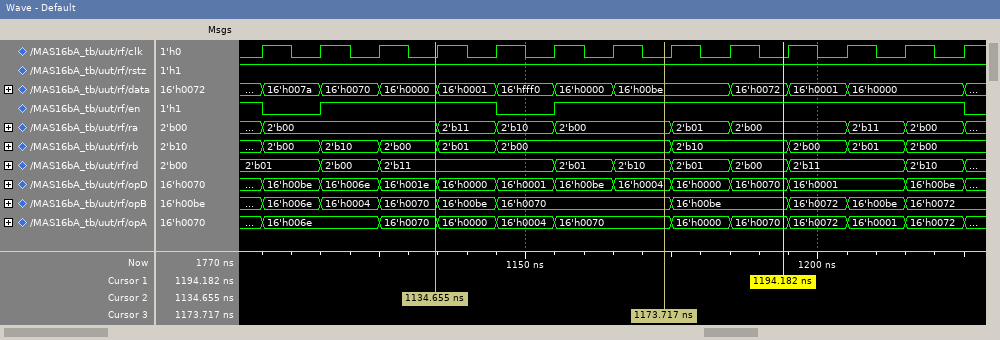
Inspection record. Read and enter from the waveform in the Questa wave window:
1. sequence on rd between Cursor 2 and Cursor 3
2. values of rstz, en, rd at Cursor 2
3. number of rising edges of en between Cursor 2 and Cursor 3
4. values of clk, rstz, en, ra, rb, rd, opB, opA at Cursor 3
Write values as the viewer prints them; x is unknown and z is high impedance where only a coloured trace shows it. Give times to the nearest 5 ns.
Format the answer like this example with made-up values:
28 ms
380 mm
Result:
2'b11, 2'b01, 2'b10
rstz=1, en=1, rd=2'b11
1
clk=0, rstz=1, en=1, ra=2'b00, rb=2'b00, rd=2'b10, opB=16'h0070, opA=16'h0070
